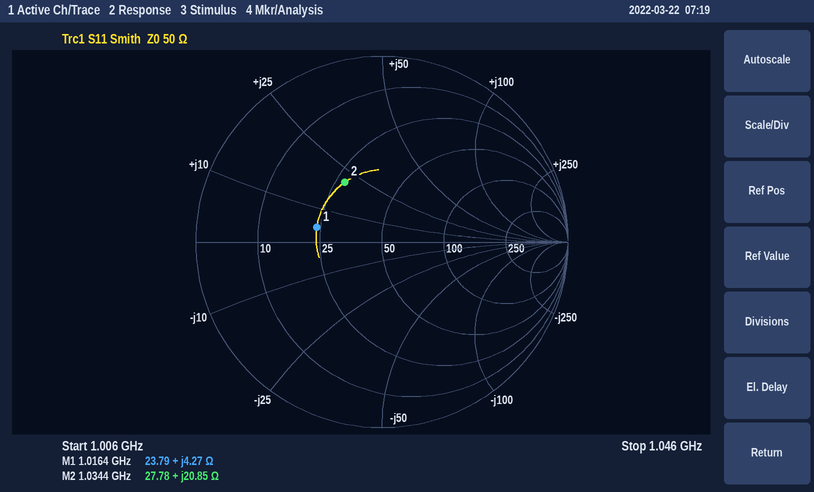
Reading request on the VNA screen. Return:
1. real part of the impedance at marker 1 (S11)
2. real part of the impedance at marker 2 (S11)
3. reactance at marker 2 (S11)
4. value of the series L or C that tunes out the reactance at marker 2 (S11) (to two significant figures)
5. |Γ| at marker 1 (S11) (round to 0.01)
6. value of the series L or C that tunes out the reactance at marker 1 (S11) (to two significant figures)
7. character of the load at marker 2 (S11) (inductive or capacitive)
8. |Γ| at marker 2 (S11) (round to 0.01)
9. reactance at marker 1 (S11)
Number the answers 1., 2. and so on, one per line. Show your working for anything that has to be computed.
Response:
1. 23.79 Ω
2. 27.78 Ω
3. +20.85 Ω
4. C = 1/(2π × 1.0344 GHz × 20.85 Ω) ≈ 7.4 pF
5. 0.36
6. C = 1/(2π × 1.0164 GHz × 4.27 Ω) ≈ 37 pF
7. inductive
8. 0.38
9. +4.27 Ω
